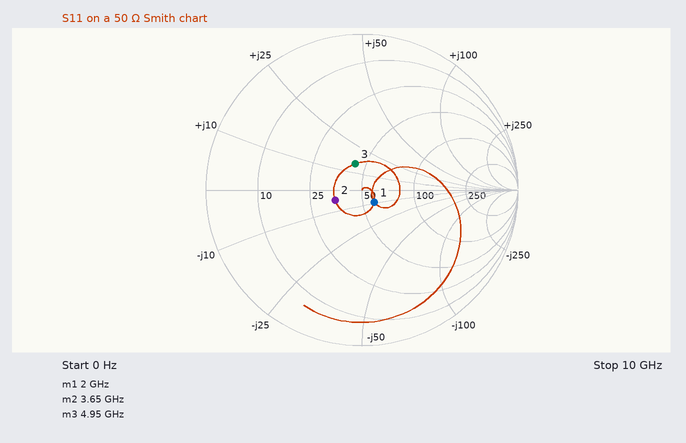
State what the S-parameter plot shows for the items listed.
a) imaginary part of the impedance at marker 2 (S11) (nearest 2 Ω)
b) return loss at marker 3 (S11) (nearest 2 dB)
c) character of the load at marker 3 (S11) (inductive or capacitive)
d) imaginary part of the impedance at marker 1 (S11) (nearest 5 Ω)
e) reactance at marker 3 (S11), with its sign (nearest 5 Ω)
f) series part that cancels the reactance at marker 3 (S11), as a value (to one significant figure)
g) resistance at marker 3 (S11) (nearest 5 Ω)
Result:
-4 Ω
16 dB
inductive
-10 Ω
+15 Ω
2 pF
45 Ω
